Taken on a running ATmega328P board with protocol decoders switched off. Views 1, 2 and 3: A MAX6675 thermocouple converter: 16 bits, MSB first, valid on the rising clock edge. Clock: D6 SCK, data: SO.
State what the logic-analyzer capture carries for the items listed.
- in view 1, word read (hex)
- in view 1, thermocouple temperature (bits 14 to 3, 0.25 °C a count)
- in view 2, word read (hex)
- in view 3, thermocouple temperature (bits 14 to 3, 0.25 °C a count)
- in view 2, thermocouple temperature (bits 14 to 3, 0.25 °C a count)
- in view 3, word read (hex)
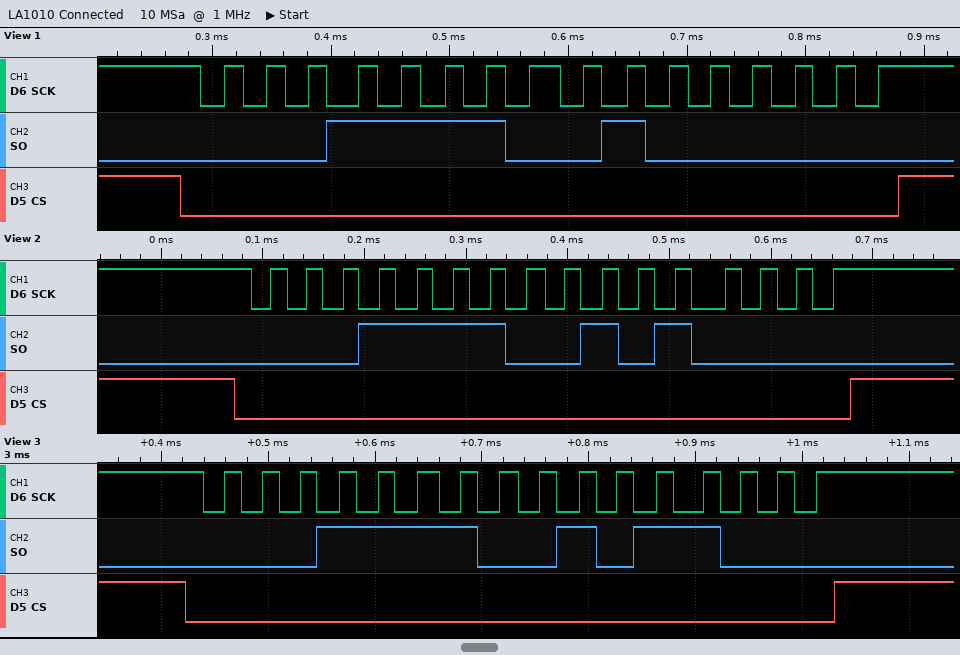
0x1E40
242.00 °C
0x1E50
242.75 °C
242.50 °C
0x1E58
